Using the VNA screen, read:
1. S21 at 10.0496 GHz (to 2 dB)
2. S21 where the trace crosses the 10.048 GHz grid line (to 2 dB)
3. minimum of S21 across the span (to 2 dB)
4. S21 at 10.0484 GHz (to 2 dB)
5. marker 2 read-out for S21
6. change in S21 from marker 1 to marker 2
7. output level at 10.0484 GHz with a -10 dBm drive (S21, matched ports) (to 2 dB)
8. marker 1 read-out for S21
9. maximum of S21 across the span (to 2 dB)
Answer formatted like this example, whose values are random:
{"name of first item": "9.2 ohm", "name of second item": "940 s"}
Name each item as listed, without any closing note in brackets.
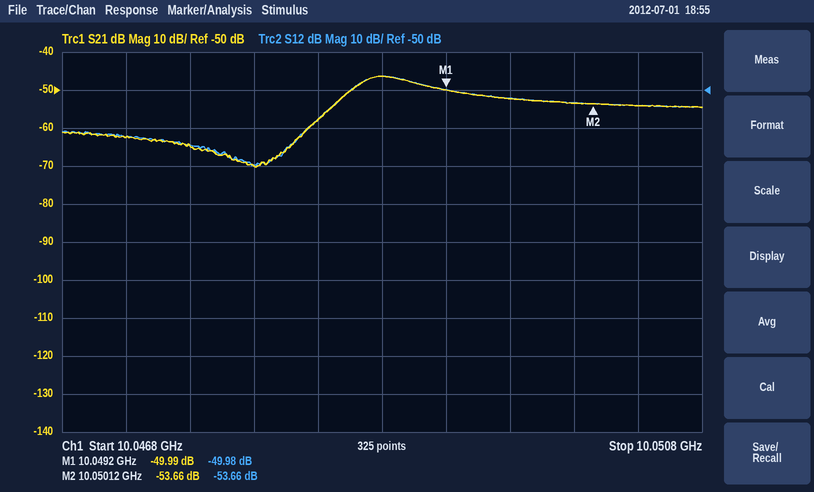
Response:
{"S21 at 10.0496 GHz": "-52 dB", "S21 where the trace crosses the 10.048 GHz grid line": "-70 dB", "minimum of S21 across the span": "-70 dB", "S21 at 10.0484 GHz": "-58 dB", "marker 2 read-out for S21": "-53.66 dB", "change in S21 from marker 1 to marker 2": "-3.67 dB", "output level at 10.0484 GHz with a -10 dBm drive (S21, matched ports)": "-68 dBm", "marker 1 read-out for S21": "-49.99 dB", "maximum of S21 across the span": "-46 dB"}
